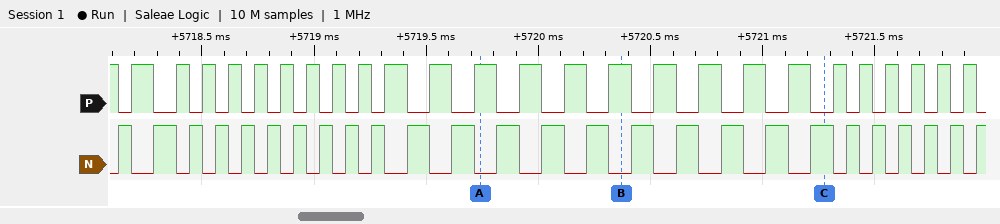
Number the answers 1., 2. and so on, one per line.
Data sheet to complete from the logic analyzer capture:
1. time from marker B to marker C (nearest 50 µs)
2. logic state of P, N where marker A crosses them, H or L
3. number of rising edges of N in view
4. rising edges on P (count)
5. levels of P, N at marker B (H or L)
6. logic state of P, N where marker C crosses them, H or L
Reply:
1. 900 µs
2. P=H, N=L
3. 26
4. 25
5. P=H, N=L
6. P=L, N=H
